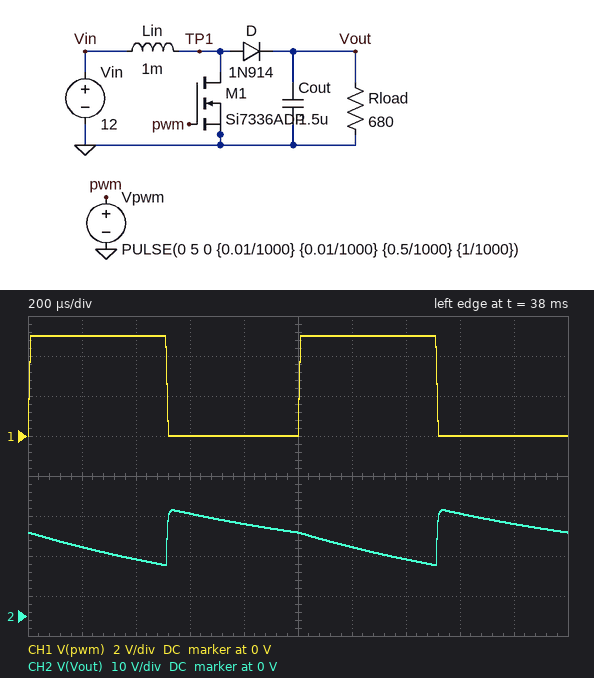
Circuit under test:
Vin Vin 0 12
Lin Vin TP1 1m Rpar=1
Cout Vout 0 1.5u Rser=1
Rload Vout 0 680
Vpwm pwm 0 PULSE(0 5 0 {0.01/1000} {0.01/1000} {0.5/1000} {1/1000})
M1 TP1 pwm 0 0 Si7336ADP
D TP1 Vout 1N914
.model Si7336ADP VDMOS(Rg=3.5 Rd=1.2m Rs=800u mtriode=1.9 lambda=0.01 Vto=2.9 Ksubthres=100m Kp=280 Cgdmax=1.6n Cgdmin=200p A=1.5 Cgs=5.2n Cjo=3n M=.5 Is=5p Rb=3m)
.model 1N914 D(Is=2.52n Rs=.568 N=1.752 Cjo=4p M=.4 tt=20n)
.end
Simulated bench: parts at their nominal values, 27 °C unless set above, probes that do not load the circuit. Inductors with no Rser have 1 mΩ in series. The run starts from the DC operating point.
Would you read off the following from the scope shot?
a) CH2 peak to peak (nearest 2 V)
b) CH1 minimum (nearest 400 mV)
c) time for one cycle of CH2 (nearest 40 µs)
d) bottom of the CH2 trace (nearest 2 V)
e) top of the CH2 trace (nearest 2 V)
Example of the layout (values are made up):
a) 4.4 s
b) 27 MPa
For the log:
a) 14 V
b) 0 V
c) 1.00 ms
d) 12 V
e) 26 V
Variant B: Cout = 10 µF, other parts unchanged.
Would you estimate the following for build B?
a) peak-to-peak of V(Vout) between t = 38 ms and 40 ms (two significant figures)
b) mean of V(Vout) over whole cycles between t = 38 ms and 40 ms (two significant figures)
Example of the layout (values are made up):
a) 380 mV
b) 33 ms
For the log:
a) 3.3 V
b) 24 V
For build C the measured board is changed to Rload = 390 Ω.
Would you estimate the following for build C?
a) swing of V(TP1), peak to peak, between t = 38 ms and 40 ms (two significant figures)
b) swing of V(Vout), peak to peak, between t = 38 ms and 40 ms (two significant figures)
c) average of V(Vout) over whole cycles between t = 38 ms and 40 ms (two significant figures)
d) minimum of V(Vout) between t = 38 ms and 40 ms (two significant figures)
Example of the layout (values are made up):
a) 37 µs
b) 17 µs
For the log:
a) 27 V
b) 18 V
c) 19 V
d) 8.7 V
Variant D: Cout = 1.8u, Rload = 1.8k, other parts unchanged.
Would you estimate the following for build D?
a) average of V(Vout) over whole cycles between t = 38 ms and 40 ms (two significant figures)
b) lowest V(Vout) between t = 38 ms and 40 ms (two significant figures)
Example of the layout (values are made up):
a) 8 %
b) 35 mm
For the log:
a) 23 V
b) 20 V
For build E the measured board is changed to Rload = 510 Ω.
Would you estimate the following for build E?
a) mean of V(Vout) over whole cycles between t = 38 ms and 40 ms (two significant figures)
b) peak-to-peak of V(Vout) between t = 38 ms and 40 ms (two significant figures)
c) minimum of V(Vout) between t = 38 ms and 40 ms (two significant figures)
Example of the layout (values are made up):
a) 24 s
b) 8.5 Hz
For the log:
a) 19 V
b) 16 V
c) 11 V
